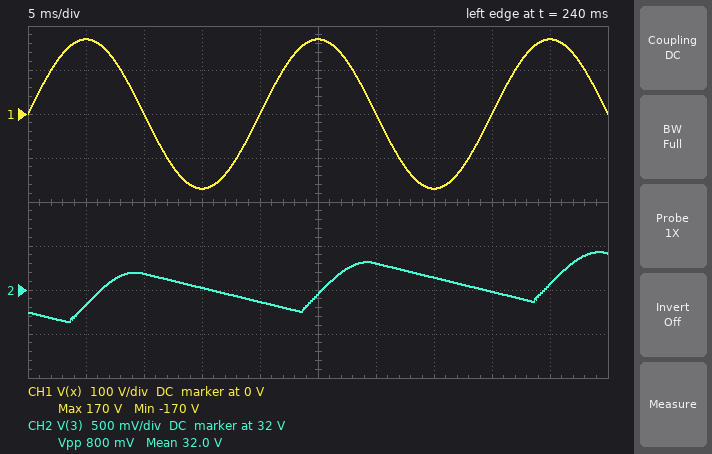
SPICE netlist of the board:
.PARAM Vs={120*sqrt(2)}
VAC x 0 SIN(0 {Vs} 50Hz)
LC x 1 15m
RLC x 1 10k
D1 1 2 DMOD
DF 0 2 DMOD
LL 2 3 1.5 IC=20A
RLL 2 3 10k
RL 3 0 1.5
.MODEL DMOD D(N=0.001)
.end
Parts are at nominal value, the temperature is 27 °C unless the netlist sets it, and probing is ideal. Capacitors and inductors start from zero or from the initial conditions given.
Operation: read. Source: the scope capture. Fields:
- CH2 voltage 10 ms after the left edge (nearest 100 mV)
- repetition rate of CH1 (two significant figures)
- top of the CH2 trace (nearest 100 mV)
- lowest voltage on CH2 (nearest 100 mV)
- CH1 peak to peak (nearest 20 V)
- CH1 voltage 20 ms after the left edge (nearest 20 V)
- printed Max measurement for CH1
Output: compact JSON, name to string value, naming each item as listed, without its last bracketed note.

{"CH2 voltage 10 ms after the left edge": "32.2 V", "repetition rate of CH1": "50 Hz", "top of the CH2 trace": "32.4 V", "lowest voltage on CH2": "31.6 V", "CH1 peak to peak": "340 V", "CH1 voltage 20 ms after the left edge": "0 V", "printed Max measurement for CH1": "170 V"}
